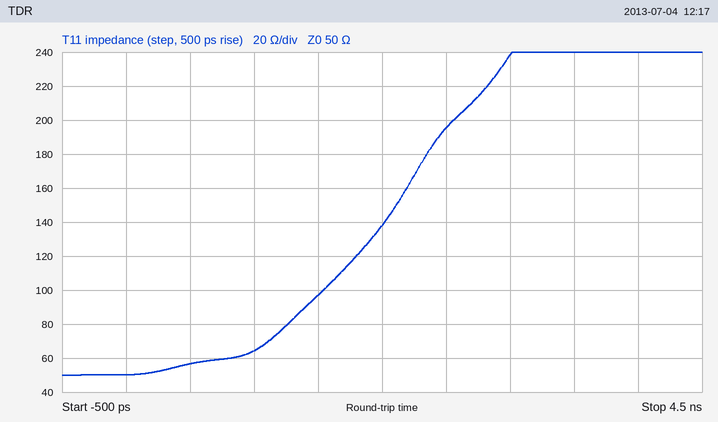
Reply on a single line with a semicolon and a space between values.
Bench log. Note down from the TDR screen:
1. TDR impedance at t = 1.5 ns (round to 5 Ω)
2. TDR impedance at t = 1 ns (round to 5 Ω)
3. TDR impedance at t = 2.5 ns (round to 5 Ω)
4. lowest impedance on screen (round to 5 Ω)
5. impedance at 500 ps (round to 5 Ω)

95 Ω; 65 Ω; 195 Ω; 50 Ω; 55 Ω
